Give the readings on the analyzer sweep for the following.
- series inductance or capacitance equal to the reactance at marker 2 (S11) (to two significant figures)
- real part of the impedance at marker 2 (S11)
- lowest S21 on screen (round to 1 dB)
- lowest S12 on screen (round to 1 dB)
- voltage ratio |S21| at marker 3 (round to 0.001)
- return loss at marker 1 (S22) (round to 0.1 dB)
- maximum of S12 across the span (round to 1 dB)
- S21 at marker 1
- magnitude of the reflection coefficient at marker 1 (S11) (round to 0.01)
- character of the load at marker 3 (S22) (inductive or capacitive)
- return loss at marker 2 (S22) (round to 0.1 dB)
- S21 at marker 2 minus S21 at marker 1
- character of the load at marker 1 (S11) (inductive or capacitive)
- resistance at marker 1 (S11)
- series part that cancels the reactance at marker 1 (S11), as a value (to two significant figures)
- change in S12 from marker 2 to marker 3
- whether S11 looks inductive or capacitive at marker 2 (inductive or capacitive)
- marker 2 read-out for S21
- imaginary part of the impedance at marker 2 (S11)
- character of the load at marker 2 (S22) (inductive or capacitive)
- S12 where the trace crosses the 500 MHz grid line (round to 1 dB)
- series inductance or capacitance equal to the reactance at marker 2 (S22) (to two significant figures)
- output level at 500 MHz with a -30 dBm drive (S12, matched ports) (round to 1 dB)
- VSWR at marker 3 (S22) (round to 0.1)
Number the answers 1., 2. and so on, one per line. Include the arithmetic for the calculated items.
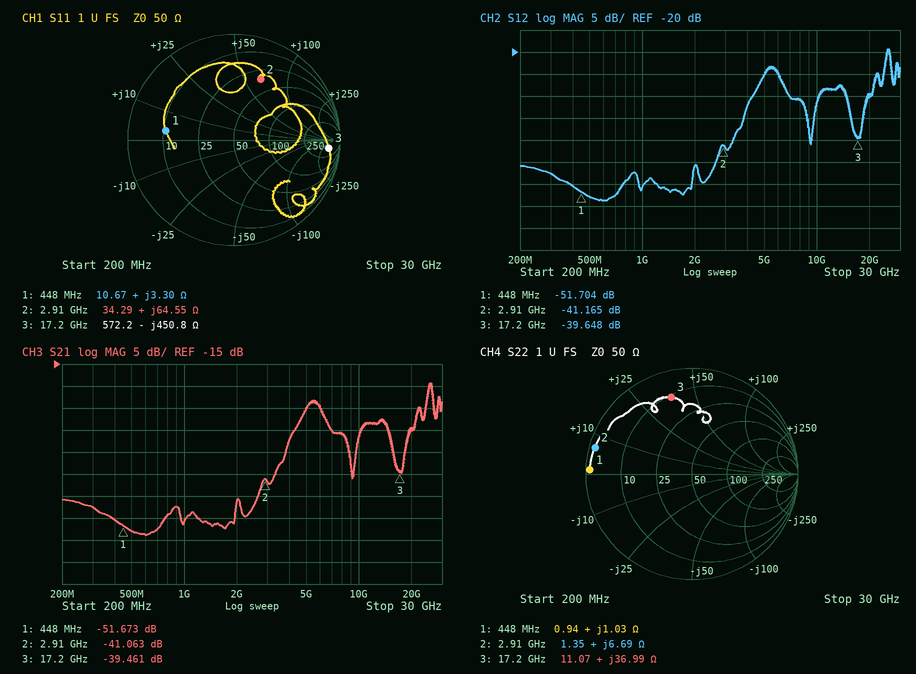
1. L = 64.55 Ω/(2π × 2.91 GHz) ≈ 3.5 nH
2. 34.29 Ω
3. -54 dB
4. -54 dB
5. 10^(-39.461/20) ≈ 0.011
6. 0.3 dB
7. -19 dB
8. -51.673 dB
9. 0.65
10. inductive
11. 0.5 dB
12. -41.063 − (-51.673) = 10.610 dB
13. inductive
14. 10.67 Ω
15. C = 1/(2π × 448 MHz × 3.3 Ω) ≈ 108 pF, so 110 pF to two significant figures
16. -39.648 − (-41.165) = 1.517 dB
17. inductive
18. -41.063 dB
19. +64.55 Ω
20. inductive
21. -53 dB
22. L = 6.69 Ω/(2π × 2.91 GHz) ≈ 366 pH, so 370 pH to two significant figures
23. -30 dBm + (-53 dB) = -83 dBm
24. 7.1
